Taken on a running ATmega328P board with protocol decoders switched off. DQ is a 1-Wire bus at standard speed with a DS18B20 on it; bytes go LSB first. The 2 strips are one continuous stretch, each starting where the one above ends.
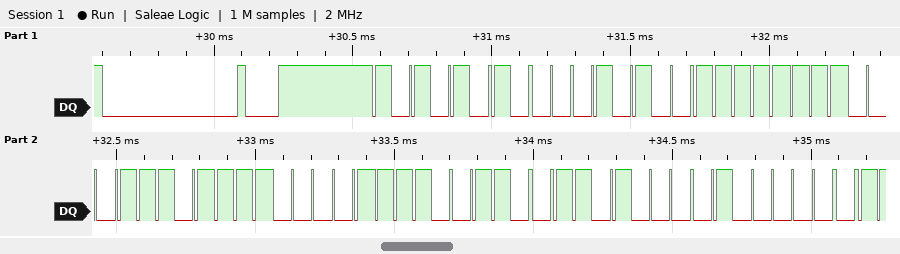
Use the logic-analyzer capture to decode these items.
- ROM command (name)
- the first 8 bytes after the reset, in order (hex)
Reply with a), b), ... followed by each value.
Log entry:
a) Match ROM
b) 55 28 FF B8 87 67 16 02
